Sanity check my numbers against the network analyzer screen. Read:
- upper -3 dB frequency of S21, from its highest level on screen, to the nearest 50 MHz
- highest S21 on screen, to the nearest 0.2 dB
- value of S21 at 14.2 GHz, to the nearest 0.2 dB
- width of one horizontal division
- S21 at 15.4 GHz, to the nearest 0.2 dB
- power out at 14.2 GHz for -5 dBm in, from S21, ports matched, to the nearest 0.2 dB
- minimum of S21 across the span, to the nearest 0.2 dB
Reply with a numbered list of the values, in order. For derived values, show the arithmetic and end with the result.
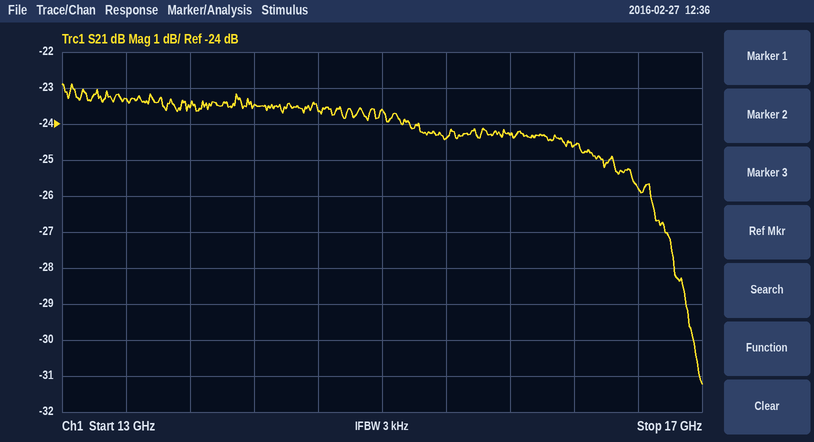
1. 16.60 GHz
2. -22.8 dB
3. -23.4 dB
4. 400 MHz
5. -24.4 dB
6. -5 dBm + (-23.4 dB) = -28.4 dBm
7. -31.2 dB
